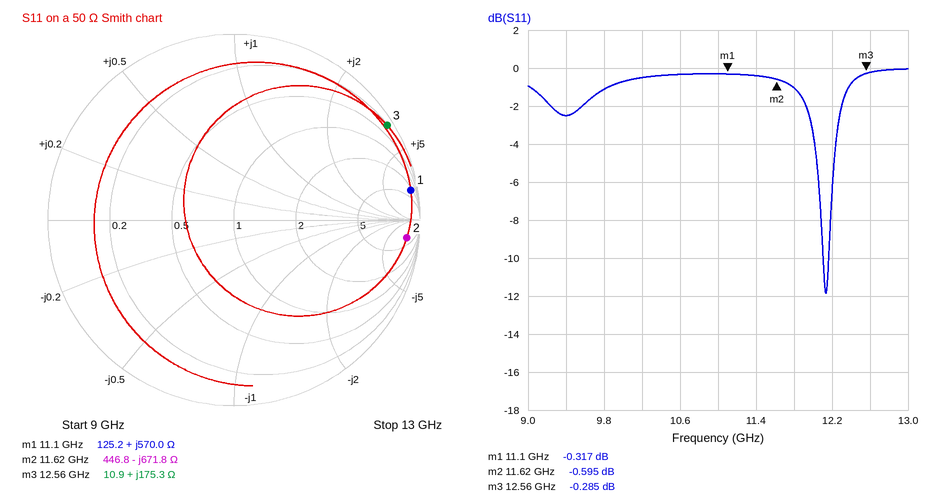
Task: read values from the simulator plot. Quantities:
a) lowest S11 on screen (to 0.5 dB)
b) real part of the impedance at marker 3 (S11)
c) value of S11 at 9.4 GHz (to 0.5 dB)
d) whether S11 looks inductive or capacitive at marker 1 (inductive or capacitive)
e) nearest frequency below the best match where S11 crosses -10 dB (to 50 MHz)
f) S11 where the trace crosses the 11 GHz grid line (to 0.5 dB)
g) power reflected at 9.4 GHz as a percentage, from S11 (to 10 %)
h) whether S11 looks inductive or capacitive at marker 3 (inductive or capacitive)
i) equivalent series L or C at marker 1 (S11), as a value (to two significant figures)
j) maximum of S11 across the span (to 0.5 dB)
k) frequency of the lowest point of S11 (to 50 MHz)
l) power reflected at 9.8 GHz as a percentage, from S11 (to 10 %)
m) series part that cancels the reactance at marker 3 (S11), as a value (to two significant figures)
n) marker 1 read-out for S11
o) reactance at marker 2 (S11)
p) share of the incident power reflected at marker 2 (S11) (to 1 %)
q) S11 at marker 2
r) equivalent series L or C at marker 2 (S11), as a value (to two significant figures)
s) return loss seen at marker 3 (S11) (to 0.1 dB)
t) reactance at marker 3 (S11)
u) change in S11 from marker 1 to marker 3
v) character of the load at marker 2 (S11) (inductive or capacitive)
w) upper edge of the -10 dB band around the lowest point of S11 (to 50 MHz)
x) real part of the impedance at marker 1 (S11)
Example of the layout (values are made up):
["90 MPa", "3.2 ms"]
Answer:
["-12.0 dB", "10.9 Ω", "-2.5 dB", "inductive", "12.10 GHz", "-0.5 dB", "60 %", "inductive", "8.2 nH", "0.0 dB", "12.15 GHz", "80 %", "72 fF", "-0.317 dB", "-671.8 Ω", "87 %", "-0.595 dB", "20 fF", "0.3 dB", "+175.3 Ω", "0.032 dB", "capacitive", "12.15 GHz", "125.2 Ω"]
